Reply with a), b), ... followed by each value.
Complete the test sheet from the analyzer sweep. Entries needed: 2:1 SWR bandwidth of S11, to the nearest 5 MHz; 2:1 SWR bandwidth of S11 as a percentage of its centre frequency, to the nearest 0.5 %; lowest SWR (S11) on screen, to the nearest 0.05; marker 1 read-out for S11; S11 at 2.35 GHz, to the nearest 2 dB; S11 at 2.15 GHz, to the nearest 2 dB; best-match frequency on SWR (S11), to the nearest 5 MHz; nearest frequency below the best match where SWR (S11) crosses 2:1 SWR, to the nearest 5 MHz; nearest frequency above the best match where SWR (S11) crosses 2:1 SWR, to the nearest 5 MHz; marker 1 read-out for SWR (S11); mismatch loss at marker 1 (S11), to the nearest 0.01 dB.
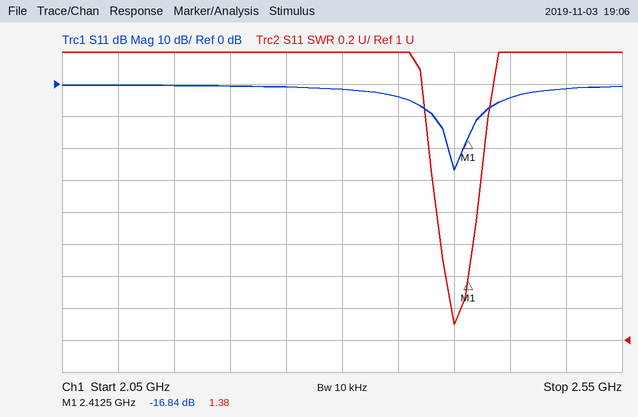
a) 45 MHz
b) 2.0 %
c) 1.10
d) -16.84 dB
e) -4 dB
f) 0 dB
g) 2.400 GHz
h) 2.380 GHz
i) 2.425 GHz
j) 1.38
k) 0.09 dB
